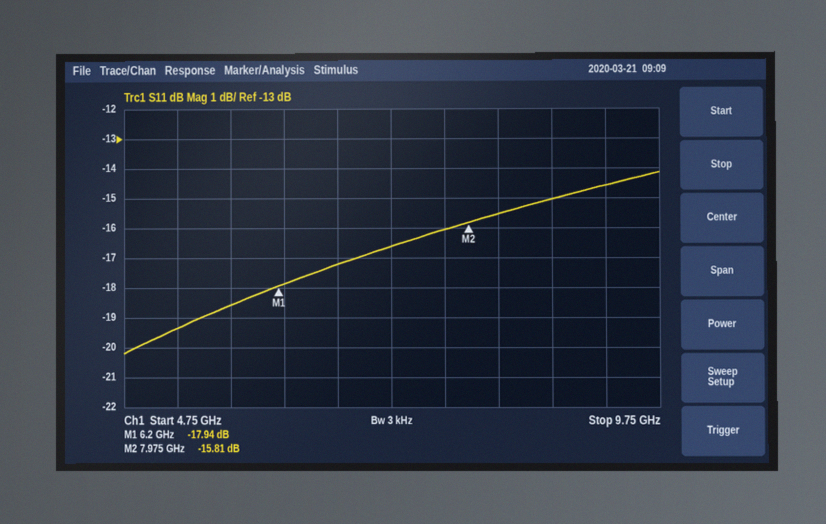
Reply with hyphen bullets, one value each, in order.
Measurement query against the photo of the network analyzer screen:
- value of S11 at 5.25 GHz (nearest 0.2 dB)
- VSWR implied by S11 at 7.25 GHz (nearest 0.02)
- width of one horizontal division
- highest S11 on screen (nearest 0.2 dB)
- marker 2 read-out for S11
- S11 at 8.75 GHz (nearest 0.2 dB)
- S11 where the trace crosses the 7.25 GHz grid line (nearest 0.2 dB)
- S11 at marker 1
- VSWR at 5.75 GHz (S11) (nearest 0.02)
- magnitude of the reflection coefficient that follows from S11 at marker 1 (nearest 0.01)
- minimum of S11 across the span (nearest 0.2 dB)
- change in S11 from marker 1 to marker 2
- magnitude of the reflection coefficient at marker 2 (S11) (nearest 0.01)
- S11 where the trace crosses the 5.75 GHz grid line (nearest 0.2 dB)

- -19.4 dB
- 1.34
- 500 MHz
- -14.2 dB
- -15.81 dB
- -15.0 dB
- -16.6 dB
- -17.94 dB
- 1.26
- 0.13
- -20.2 dB
- 2.13 dB
- 0.16
- -18.6 dB
